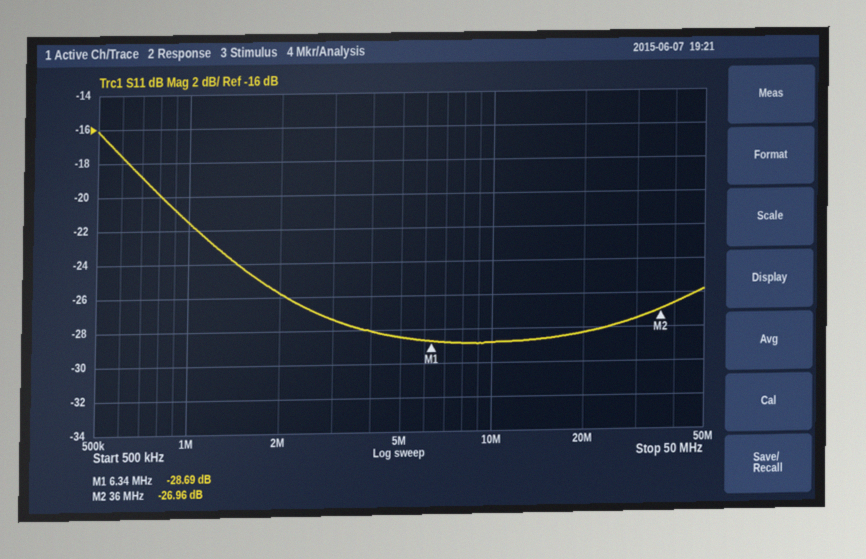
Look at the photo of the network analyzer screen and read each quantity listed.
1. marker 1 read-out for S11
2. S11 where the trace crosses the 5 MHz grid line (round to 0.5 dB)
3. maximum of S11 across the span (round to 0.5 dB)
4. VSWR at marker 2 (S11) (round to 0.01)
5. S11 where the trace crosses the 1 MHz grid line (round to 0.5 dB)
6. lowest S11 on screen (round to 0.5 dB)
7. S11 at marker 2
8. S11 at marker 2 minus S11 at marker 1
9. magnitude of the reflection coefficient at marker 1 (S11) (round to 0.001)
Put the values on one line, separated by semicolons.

-28.69 dB; -28.5 dB; -16.0 dB; 1.09; -21.5 dB; -29.0 dB; -26.96 dB; 1.73 dB; 0.037
